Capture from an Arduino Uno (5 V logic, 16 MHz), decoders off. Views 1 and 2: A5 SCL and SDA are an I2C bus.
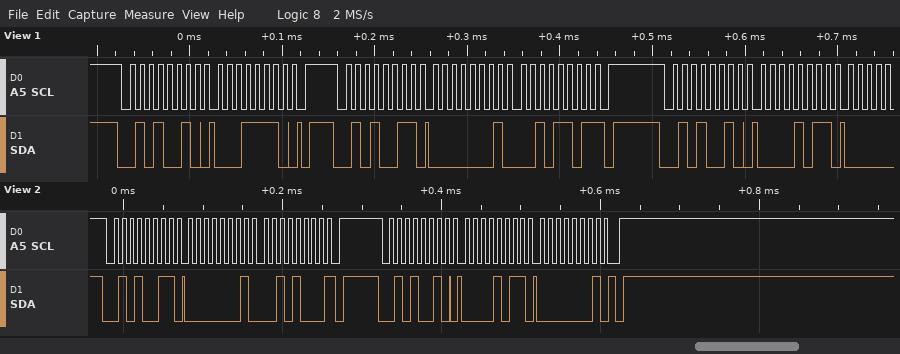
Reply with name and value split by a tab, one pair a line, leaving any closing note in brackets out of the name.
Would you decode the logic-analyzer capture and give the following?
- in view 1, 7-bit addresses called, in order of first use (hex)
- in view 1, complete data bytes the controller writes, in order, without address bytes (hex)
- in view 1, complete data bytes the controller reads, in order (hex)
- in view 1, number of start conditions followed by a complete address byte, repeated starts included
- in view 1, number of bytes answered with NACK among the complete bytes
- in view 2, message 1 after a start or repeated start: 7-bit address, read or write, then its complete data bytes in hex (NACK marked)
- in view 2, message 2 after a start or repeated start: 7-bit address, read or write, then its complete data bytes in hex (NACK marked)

in view 1, 7-bit addresses called, in order of first use	0x29
in view 1, complete data bytes the controller writes, in order, without address bytes	1E 0B
in view 1, complete data bytes the controller reads, in order	01 2D
in view 1, number of start conditions followed by a complete address byte, repeated starts included	3
in view 1, number of bytes answered with NACK among the complete bytes	1
in view 2, message 1 after a start or repeated start: 7-bit address, read or write, then its complete data bytes in hex	0x29 read: 01 28 NACK
in view 2, message 2 after a start or repeated start: 7-bit address, read or write, then its complete data bytes in hex	0x29 write: 0B 01
